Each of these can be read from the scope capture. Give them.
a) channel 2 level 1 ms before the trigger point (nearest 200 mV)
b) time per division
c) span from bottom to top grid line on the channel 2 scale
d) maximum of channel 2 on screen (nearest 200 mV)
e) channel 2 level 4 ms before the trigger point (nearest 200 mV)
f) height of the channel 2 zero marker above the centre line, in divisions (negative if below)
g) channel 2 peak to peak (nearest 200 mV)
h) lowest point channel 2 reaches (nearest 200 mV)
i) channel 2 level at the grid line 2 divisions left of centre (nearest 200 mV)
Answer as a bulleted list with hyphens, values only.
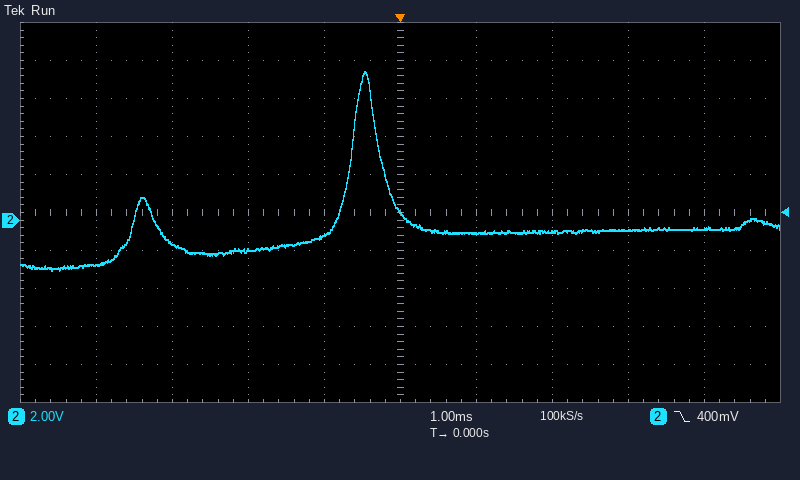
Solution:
- -800 mV
- 1 ms
- 20 V
- 7.8 V
- -2.4 V
- -0.2 div
- 10.4 V
- -2.6 V
- -1.6 V
